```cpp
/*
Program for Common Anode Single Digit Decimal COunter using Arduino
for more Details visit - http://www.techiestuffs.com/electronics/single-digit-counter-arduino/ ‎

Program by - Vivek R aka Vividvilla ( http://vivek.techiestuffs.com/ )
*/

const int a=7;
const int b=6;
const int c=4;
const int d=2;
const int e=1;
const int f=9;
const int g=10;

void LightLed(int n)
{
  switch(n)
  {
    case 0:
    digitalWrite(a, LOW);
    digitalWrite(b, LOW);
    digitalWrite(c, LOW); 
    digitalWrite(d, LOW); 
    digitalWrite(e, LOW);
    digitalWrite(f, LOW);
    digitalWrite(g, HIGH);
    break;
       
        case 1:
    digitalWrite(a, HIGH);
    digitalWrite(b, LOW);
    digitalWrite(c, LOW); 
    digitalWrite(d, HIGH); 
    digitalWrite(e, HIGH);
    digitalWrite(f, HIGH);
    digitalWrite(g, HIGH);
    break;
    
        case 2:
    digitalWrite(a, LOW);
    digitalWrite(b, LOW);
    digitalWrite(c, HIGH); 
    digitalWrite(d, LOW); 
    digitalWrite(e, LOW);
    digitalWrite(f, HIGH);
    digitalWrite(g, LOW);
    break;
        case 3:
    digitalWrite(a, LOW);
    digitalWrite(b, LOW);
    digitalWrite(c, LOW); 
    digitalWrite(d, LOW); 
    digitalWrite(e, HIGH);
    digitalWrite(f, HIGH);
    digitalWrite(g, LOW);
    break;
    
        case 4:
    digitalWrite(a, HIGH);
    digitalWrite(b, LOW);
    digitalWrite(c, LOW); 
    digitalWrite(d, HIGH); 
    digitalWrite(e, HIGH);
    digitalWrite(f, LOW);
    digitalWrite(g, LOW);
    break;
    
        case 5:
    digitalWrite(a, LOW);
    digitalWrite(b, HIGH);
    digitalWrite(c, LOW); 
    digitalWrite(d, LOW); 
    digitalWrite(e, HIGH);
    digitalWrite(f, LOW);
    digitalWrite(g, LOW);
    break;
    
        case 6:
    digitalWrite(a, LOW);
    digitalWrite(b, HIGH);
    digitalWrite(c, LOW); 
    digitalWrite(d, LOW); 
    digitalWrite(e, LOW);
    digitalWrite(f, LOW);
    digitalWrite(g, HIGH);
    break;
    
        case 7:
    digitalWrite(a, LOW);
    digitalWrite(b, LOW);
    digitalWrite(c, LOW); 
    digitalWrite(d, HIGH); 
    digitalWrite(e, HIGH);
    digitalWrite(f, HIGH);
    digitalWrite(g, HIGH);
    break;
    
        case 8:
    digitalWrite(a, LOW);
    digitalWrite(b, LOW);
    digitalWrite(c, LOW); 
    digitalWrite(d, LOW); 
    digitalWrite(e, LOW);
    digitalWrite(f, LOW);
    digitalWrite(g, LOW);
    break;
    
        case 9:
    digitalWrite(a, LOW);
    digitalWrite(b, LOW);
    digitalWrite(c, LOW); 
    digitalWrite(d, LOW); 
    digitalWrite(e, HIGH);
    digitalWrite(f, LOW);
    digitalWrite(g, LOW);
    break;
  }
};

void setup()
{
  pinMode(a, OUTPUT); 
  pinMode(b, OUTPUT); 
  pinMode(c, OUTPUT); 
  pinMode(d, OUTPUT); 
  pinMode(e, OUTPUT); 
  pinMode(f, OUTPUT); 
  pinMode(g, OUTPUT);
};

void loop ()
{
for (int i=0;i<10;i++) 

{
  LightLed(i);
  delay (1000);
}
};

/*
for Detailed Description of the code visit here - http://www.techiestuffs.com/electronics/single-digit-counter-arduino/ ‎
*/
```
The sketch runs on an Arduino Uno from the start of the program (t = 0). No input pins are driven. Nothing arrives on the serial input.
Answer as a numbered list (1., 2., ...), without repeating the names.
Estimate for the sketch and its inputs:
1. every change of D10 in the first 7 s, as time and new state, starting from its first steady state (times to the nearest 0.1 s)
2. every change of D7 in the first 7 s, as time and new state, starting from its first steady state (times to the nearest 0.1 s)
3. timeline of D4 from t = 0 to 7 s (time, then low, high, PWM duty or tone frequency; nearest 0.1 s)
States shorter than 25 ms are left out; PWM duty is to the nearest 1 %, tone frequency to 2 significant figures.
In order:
1. 0 s high; 2 s low; 6 s high
2. 0 s low; 1 s high; 2 s low; 4 s high; 5 s low
3. 0 s low; 2 s high; 3 s low
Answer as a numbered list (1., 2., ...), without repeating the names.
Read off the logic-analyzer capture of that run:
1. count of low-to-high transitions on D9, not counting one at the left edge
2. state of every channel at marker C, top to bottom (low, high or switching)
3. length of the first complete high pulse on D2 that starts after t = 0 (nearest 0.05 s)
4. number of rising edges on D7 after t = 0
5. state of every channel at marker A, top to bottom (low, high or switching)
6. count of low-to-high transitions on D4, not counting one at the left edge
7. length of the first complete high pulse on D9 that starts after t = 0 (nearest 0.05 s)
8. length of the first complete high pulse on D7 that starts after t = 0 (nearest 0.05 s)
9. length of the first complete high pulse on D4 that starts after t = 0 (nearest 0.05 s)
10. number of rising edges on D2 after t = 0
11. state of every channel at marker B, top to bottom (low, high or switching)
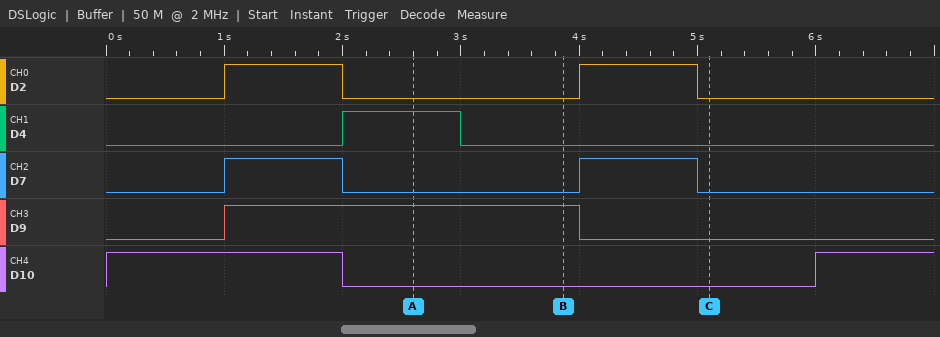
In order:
1. 1
2. D2 low, D4 low, D7 low, D9 low, D10 low
3. 1.00 s
4. 2
5. D2 low, D4 high, D7 low, D9 high, D10 low
6. 1
7. 3.00 s
8. 1.00 s
9. 1.00 s
10. 2
11. D2 low, D4 low, D7 low, D9 high, D10 low
